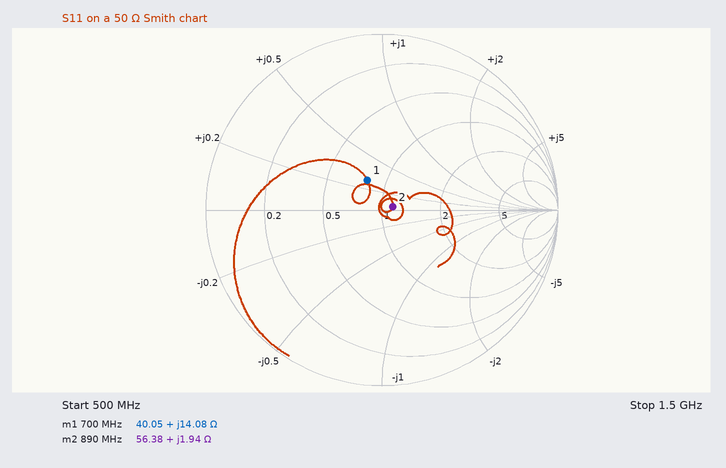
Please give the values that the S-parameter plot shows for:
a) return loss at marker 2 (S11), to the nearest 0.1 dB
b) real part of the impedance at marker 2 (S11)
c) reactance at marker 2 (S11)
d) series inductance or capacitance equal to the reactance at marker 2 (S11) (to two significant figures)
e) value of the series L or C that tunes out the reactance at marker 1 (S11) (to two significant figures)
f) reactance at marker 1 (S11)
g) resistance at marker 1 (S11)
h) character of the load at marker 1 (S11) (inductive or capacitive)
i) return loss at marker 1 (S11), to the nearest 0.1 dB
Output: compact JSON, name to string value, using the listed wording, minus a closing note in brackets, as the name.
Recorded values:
{"return loss at marker 2 (S11), to the nearest 0.1 dB": "24.1 dB", "real part of the impedance at marker 2": "56.38 Ω", "reactance at marker 2": "+1.94 Ω", "series inductance or capacitance equal to the reactance at marker 2 (S11)": "350 pH", "value of the series L or C that tunes out the reactance at marker 1 (S11)": "16 pF", "reactance at marker 1": "+14.08 Ω", "resistance at marker 1": "40.05 Ω", "character of the load at marker 1 (S11)": "inductive", "return loss at marker 1 (S11), to the nearest 0.1 dB": "14.5 dB"}
